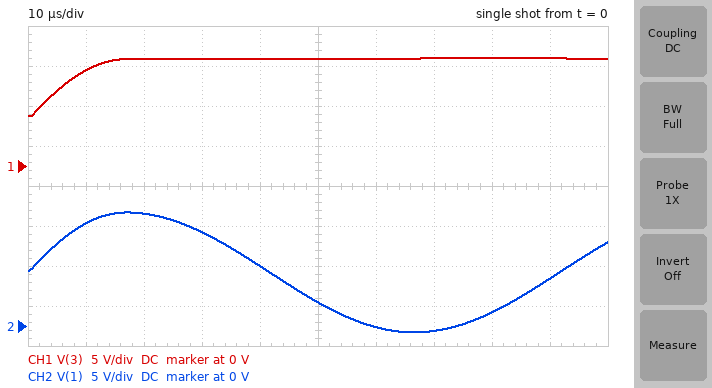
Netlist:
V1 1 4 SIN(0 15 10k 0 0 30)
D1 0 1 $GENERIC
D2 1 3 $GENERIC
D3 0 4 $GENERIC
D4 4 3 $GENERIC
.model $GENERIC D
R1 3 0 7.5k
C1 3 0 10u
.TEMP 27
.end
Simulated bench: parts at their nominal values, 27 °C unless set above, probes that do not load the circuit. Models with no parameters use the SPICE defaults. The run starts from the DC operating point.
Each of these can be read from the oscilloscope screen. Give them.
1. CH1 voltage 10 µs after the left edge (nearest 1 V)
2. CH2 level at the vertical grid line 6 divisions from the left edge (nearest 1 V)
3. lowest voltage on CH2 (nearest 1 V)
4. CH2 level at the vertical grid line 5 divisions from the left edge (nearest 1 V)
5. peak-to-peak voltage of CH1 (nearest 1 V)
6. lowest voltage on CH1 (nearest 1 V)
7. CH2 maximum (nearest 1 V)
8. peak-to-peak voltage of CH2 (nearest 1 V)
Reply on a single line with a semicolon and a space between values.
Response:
12 V; 0 V; -1 V; 3 V; 7 V; 6 V; 14 V; 15 V
